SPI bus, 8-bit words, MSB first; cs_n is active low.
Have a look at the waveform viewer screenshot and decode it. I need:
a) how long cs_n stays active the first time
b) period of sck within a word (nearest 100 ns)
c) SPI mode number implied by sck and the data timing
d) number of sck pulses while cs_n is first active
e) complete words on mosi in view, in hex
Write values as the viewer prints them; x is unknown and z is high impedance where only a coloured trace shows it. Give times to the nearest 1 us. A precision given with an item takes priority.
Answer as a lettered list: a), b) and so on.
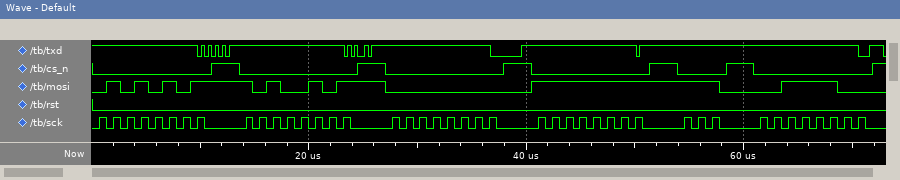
a) 11 us
b) 1300 ns
c) 0
d) 8
e) 55, A5, 00, FF, 3C
